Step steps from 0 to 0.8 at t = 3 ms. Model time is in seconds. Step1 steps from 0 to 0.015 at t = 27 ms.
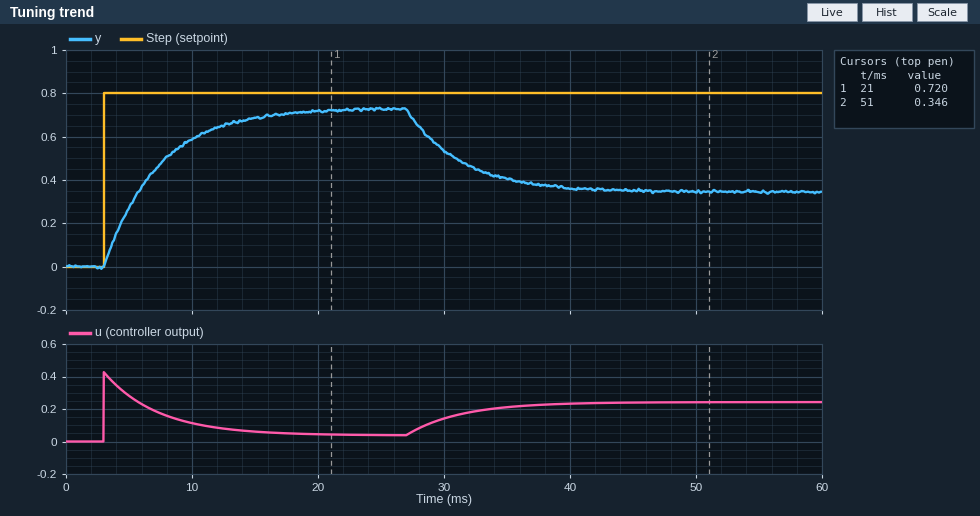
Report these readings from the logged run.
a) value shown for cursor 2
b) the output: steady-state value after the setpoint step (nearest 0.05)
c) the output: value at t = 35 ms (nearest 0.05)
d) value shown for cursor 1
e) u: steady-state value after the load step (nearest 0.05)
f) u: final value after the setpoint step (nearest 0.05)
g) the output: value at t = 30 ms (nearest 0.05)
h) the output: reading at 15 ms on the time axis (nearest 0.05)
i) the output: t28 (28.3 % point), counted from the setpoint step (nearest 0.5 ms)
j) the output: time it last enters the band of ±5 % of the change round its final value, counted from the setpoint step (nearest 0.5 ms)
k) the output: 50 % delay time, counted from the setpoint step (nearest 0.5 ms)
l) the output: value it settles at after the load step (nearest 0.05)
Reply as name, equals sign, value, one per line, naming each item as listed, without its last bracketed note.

value shown for cursor 2 = 0.346
the output: steady-state value after the setpoint step = 0.75
the output: value at t = 35 ms = 0.40
value shown for cursor 1 = 0.720
u: steady-state value after the load step = 0.25
u: final value after the setpoint step = 0.05
the output: value at t = 30 ms = 0.55
the output: reading at 15 ms on the time axis = 0.70
the output: t28 (28.3 % point), counted from the setpoint step = 1.5 ms
the output: time it last enters the band of ±5 % of the change round its final value, counted from the setpoint step = 13.0 ms
the output: 50 % delay time, counted from the setpoint step = 3.0 ms
the output: value it settles at after the load step = 0.35
